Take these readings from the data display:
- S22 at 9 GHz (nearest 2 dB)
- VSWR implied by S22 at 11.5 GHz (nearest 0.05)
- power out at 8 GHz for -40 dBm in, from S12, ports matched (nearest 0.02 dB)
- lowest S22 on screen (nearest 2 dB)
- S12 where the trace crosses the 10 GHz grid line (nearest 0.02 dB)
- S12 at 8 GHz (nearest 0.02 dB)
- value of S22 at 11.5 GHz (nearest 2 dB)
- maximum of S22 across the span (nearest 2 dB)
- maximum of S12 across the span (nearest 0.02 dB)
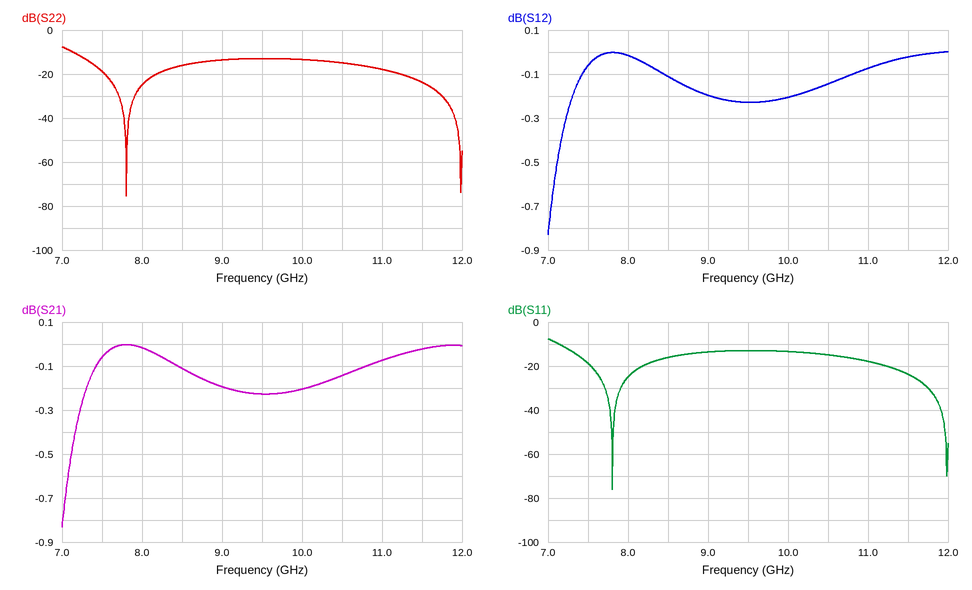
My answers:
-14 dB
1.15
-40.02 dBm
-76 dB
-0.20 dB
-0.02 dB
-24 dB
-8 dB
0.00 dB
